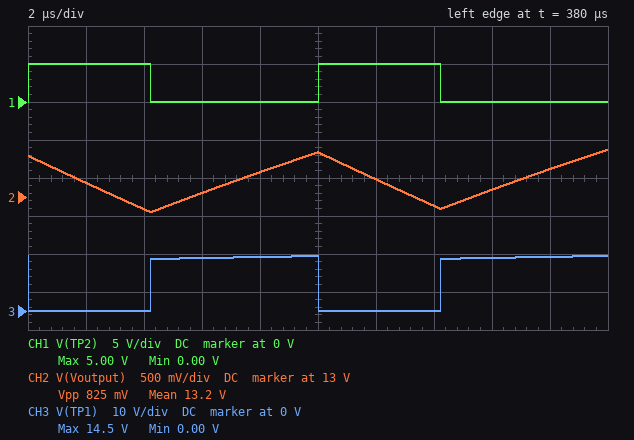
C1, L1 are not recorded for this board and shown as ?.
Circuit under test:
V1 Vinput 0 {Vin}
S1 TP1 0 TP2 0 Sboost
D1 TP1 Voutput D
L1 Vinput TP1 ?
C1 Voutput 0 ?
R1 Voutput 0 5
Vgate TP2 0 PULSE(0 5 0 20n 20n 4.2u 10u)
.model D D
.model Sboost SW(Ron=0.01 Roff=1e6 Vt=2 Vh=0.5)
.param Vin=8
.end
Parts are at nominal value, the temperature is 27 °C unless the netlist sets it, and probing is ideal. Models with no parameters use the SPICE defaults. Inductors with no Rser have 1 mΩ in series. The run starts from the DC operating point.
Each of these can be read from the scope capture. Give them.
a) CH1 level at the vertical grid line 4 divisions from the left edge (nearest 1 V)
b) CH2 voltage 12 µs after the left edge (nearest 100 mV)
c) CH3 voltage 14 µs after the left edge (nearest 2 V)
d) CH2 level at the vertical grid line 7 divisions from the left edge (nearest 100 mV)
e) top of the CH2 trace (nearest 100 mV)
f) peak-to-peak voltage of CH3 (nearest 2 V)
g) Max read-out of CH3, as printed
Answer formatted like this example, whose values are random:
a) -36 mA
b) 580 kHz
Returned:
a) 0 V
b) 13.2 V
c) 0 V
d) 12.9 V
e) 13.6 V
f) 14 V
g) 14.5 V
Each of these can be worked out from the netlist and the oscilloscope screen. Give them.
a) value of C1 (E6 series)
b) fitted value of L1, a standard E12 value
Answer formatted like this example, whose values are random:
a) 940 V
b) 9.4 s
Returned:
a) 15 µF
b) 220 µH
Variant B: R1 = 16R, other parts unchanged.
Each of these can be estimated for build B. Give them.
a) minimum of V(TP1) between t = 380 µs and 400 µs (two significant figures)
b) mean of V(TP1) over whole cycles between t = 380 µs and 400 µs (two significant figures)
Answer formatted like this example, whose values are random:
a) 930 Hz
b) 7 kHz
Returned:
a) 12 mV
b) 9.5 V
